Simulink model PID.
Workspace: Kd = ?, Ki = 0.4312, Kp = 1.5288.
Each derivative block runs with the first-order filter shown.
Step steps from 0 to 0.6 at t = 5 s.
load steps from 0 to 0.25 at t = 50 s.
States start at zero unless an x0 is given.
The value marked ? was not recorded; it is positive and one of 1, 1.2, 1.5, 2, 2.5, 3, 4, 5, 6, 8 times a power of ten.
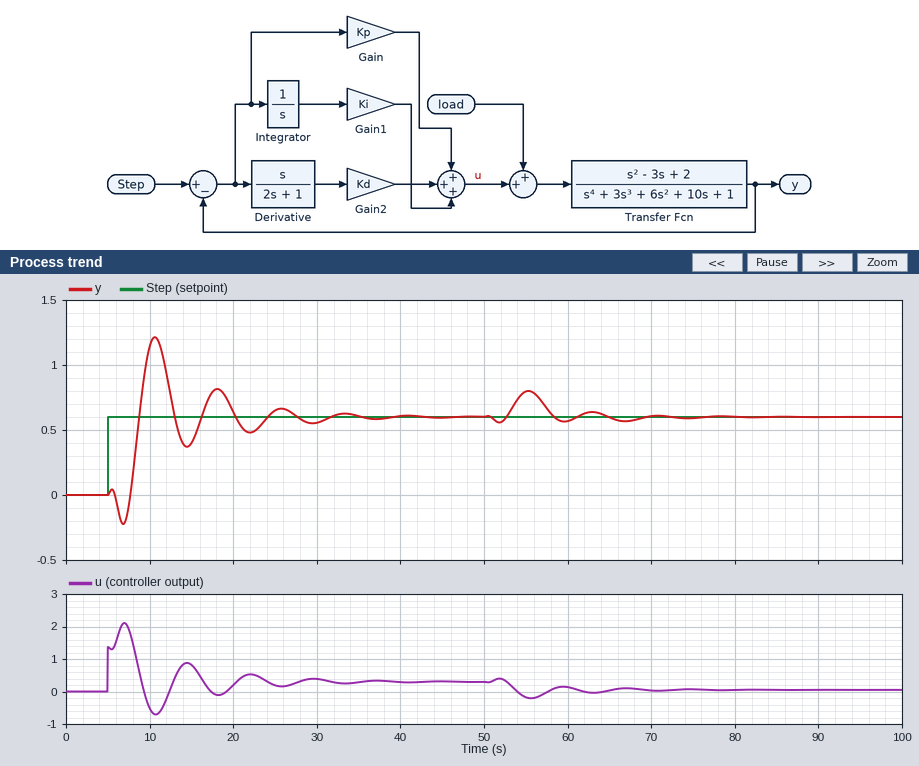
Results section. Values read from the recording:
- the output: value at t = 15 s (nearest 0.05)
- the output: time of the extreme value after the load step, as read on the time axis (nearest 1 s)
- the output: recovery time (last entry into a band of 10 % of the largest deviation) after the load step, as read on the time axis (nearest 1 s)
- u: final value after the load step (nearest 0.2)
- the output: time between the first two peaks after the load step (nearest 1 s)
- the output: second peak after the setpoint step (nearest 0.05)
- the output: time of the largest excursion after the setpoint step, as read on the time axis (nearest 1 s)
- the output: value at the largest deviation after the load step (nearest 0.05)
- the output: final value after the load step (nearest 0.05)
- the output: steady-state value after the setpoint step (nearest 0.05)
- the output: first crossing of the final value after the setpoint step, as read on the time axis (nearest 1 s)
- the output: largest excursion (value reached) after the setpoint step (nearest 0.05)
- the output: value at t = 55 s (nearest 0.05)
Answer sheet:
0.40
55 s
68 s
0.0
8 s
0.80
11 s
0.80
0.60
0.60
9 s
1.20
0.80
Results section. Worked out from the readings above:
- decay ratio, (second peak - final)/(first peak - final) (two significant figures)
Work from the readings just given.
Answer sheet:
0.33
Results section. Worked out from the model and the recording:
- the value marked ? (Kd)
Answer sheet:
1.5
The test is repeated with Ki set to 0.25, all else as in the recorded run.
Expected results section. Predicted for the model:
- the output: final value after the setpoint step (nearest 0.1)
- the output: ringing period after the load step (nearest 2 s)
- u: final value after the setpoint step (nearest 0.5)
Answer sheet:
0.6
6 s
0.5
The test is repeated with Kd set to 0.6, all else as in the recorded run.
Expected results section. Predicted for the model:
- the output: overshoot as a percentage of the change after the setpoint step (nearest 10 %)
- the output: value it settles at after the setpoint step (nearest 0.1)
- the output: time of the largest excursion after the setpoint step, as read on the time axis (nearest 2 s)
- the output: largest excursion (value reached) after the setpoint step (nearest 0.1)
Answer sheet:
90 %
0.6
12 s
1.1
